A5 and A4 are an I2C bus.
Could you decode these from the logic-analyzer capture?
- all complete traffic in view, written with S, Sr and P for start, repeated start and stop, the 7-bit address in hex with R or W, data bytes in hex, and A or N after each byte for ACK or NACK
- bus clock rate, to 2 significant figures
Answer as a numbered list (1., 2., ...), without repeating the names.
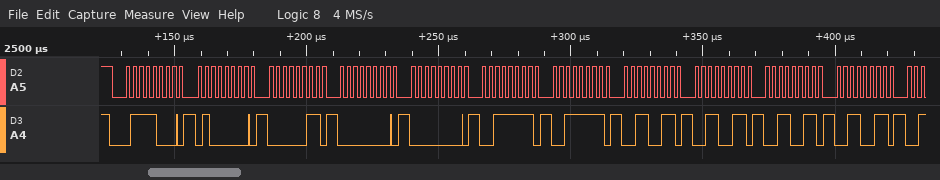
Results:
1. S 3CW A 40 A 03 A 00 A 00 A 3F A 3F A 33 A 33 A 33 A 33 A
2. 400 kHz
